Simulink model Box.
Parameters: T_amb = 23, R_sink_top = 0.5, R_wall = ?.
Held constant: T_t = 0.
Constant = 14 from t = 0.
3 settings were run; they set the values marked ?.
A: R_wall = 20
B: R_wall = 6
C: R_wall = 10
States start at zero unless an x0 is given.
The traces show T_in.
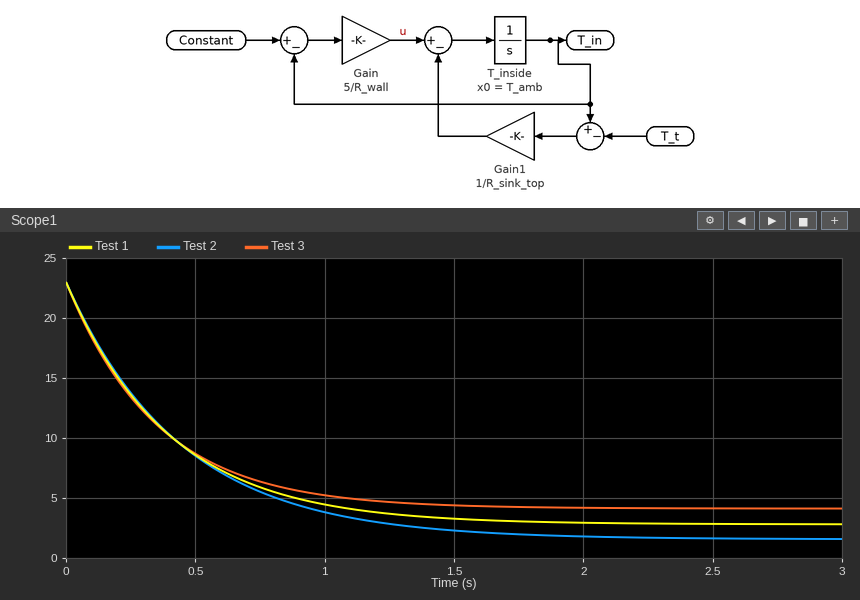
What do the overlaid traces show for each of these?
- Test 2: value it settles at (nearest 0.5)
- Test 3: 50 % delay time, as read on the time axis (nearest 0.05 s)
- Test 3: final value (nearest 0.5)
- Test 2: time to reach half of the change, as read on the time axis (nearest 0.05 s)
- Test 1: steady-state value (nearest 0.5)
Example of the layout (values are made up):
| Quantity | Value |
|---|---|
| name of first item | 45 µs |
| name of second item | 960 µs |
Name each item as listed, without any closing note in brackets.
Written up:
| Quantity | Value |
|---|---|
| Test 2: value it settles at | 1.5 |
| Test 3: 50 % delay time, as read on the time axis | 0.25 s |
| Test 3: final value | 4.0 |
| Test 2: time to reach half of the change, as read on the time axis | 0.30 s |
| Test 1: steady-state value | 3.0 |
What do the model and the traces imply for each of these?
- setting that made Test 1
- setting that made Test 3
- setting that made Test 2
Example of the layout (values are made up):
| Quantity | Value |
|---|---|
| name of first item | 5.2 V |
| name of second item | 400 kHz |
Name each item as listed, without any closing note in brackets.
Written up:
| Quantity | Value |
|---|---|
| setting that made Test 1 | C |
| setting that made Test 3 | B |
| setting that made Test 2 | A |
